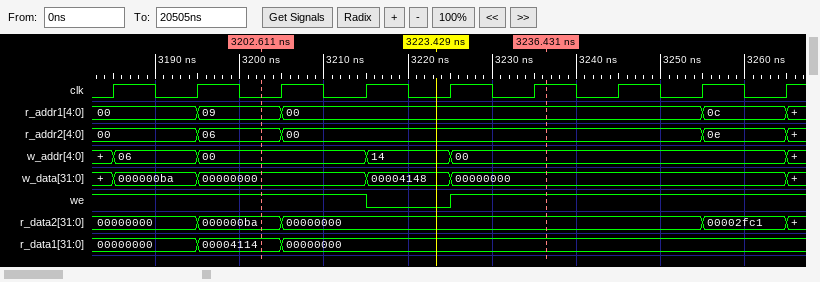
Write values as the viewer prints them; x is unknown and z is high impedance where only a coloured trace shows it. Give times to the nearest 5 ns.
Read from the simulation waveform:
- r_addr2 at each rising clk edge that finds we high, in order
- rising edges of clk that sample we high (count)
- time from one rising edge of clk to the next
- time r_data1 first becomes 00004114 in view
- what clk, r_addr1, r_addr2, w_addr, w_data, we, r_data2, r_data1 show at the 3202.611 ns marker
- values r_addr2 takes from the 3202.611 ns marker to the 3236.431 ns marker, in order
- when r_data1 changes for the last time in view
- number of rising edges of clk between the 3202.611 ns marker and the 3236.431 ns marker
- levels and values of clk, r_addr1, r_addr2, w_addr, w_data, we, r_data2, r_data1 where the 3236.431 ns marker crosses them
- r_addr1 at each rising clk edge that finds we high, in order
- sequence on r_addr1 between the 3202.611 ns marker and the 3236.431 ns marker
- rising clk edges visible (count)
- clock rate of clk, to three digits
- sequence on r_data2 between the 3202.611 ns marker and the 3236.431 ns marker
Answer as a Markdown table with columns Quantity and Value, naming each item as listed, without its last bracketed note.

| Quantity | Value |
|---|---|
| r_addr2 at each rising clk edge that finds we high, in order | 00, 00, 06, 00, 00, 00, 00, 0e |
| rising edges of clk that sample we high | 8 |
| time from one rising edge of clk to the next | 10 ns |
| time r_data1 first becomes 00004114 in view | 3195 ns |
| what clk, r_addr1, r_addr2, w_addr, w_data, we, r_data2, r_data1 show at the 3202.611 ns marker | clk=0, r_addr1=09, r_addr2=06, w_addr=00, w_data=00000000, we=1, r_data2=000000ba, r_data1=00004114 |
| values r_addr2 takes from the 3202.611 ns marker to the 3236.431 ns marker, in order | 06, 00 |
| when r_data1 changes for the last time in view | 3205 ns |
| number of rising edges of clk between the 3202.611 ns marker and the 3236.431 ns marker | 4 |
| levels and values of clk, r_addr1, r_addr2, w_addr, w_data, we, r_data2, r_data1 where the 3236.431 ns marker crosses them | clk=1, r_addr1=00, r_addr2=00, w_addr=00, w_data=00000000, we=1, r_data2=00000000, r_data1=00000000 |
| r_addr1 at each rising clk edge that finds we high, in order | 00, 00, 09, 00, 00, 00, 00, 0c |
| sequence on r_addr1 between the 3202.611 ns marker and the 3236.431 ns marker | 09, 00 |
| rising clk edges visible | 9 |
| clock rate of clk, to three digits | 100 MHz |
| sequence on r_data2 between the 3202.611 ns marker and the 3236.431 ns marker | 000000ba, 00000000 |
